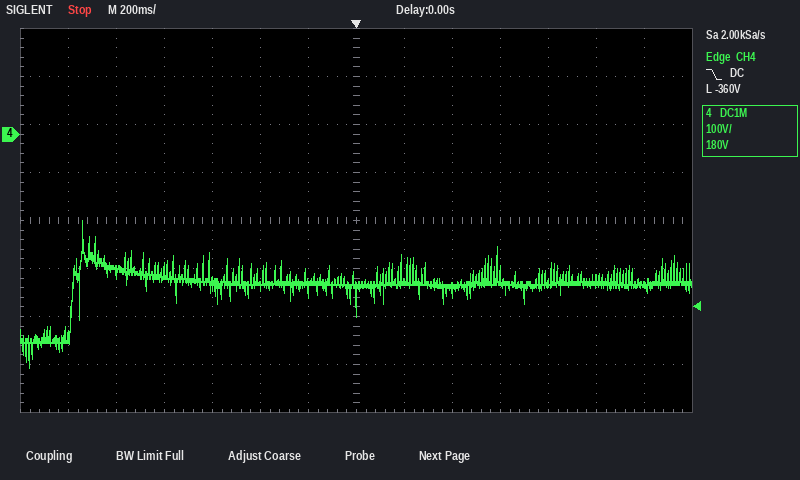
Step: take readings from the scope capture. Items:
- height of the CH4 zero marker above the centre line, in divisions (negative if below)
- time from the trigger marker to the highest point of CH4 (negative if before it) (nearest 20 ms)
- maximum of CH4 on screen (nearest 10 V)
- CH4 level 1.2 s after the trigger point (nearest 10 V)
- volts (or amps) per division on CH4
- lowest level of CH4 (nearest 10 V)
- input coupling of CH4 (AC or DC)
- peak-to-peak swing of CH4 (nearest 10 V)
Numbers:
+1.8 div
-1.14 s
-180 V
-310 V
100 V
-490 V
DC
310 V
